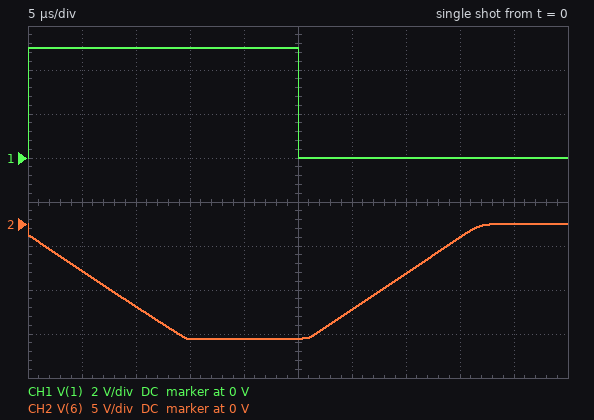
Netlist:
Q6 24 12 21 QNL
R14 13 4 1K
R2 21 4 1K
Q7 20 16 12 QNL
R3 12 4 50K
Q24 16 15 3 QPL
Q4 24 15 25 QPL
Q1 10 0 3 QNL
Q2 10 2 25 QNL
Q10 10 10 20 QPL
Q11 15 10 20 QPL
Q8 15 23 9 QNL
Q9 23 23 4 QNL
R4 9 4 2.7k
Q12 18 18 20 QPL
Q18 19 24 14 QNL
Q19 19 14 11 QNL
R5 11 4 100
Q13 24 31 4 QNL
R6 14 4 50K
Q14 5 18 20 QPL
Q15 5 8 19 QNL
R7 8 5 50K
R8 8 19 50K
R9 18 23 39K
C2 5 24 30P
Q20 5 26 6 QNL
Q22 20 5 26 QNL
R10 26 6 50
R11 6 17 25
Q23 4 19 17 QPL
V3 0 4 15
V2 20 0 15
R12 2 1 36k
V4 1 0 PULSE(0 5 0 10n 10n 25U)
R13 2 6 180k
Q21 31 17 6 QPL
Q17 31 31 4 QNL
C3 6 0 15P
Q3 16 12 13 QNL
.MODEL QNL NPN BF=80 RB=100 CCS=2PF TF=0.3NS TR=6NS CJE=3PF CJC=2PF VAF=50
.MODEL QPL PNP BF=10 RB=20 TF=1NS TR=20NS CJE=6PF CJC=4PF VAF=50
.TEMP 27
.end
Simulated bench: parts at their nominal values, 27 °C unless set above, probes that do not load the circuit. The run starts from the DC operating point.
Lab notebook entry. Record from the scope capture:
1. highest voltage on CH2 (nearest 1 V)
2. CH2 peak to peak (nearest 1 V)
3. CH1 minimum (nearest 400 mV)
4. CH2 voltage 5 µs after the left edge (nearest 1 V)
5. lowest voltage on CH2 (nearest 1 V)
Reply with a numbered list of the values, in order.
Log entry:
1. 0 V
2. 13 V
3. 0 V
4. -5 V
5. -13 V
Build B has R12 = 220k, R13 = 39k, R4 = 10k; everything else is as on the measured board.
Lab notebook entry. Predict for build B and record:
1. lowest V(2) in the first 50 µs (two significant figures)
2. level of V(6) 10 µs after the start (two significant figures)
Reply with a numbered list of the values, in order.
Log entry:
1. -650 mV
2. -880 mV
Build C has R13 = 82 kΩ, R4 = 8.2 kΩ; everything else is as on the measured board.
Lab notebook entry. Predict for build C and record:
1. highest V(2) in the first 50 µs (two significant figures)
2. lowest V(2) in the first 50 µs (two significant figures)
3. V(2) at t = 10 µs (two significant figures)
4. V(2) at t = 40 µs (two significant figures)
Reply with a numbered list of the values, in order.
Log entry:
1. 3.3 V
2. -2.7 V
3. 2.2 V
4. -1.2 V
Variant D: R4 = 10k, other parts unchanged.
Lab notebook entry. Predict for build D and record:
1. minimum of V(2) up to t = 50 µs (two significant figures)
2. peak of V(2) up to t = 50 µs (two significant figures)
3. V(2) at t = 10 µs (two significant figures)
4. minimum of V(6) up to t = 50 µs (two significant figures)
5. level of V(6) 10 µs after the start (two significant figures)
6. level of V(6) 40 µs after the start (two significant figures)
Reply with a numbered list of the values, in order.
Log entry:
1. -1.4 V
2. 4.1 V
3. 3.5 V
4. -8.3 V
5. -4.1 V
6. -4.8 V
